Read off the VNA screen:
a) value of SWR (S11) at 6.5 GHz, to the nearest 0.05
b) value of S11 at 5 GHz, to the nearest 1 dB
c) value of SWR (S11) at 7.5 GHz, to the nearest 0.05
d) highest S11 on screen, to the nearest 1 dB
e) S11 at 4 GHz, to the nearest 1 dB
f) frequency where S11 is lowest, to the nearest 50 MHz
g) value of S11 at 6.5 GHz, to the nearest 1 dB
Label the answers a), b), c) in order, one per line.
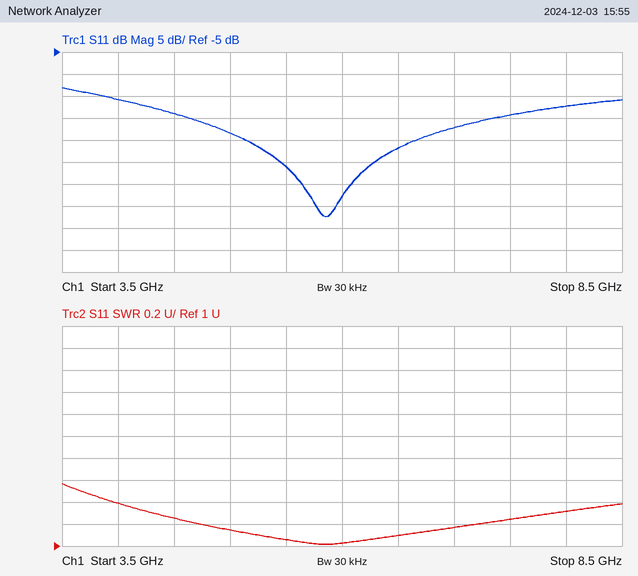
a) 1.10
b) -23 dB
c) 1.25
d) -13 dB
e) -16 dB
f) 5.85 GHz
g) -27 dB
